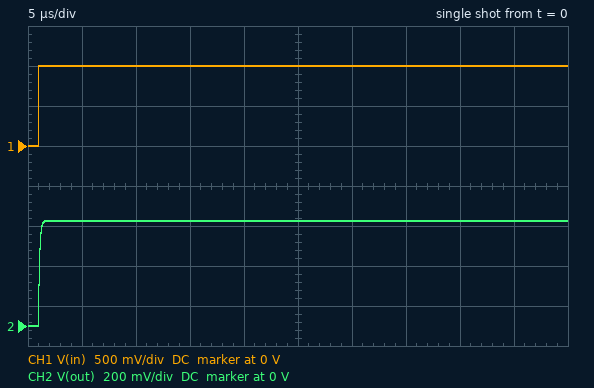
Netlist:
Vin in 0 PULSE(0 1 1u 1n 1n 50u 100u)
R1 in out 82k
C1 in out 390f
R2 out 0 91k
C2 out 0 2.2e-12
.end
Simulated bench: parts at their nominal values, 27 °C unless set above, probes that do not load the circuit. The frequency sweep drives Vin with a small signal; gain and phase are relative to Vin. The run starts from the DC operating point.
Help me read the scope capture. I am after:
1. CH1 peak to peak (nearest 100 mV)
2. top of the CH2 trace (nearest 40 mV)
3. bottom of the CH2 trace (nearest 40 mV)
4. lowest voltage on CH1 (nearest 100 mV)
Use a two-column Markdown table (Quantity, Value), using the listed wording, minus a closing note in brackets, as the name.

| Quantity | Value |
|---|---|
| CH1 peak to peak | 1.0 V |
| top of the CH2 trace | 520 mV |
| bottom of the CH2 trace | 0 V |
| lowest voltage on CH1 | 0 V |
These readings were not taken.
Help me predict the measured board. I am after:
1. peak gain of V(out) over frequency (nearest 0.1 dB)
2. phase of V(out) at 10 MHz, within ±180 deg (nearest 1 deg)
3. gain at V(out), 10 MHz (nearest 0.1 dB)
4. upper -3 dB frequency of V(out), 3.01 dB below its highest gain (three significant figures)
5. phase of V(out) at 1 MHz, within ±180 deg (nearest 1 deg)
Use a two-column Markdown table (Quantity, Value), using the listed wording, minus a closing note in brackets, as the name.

| Quantity | Value |
|---|---|
| peak gain of V(out) over frequency | -5.6 dB |
| phase of V(out) at 10 MHz, within ±180 deg | -18 deg |
| gain at V(out), 10 MHz | -15.6 dB |
| upper -3 dB frequency of V(out), 3.01 dB below its highest gain | 1.56 MHz |
| phase of V(out) at 1 MHz, within ±180 deg | -24 deg |
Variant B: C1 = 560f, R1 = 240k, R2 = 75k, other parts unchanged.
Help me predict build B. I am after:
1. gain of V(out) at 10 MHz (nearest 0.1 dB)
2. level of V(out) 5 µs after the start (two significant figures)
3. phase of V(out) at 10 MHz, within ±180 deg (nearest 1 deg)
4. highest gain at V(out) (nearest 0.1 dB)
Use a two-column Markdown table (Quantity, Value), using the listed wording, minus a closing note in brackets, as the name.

| Quantity | Value |
|---|---|
| gain of V(out) at 10 MHz | -13.8 dB |
| level of V(out) 5 µs after the start | 240 mV |
| phase of V(out) at 10 MHz, within ±180 deg | -1 deg |
| highest gain at V(out) | -12.5 dB |
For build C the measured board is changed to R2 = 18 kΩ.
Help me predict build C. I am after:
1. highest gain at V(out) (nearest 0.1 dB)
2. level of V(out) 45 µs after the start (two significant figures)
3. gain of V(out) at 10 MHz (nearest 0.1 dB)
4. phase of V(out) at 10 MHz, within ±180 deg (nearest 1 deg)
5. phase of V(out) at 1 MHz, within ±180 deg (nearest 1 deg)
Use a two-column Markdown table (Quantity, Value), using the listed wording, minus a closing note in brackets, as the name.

| Quantity | Value |
|---|---|
| highest gain at V(out) | -14.9 dB |
| level of V(out) 45 µs after the start | 180 mV |
| gain of V(out) at 10 MHz | -16.2 dB |
| phase of V(out) at 10 MHz, within ±180 deg | -4 deg |
| phase of V(out) at 1 MHz, within ±180 deg | -2 deg |
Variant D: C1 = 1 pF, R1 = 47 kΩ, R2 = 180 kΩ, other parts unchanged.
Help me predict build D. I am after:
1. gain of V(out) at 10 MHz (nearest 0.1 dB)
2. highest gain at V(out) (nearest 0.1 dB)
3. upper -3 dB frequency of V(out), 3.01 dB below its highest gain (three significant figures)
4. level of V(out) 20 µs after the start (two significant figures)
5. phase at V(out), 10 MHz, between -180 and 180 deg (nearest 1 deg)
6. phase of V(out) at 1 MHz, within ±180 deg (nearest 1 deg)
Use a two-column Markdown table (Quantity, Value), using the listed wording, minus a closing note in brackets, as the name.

| Quantity | Value |
|---|---|
| gain of V(out) at 10 MHz | -9.7 dB |
| highest gain at V(out) | -2.0 dB |
| upper -3 dB frequency of V(out), 3.01 dB below its highest gain | 1.61 MHz |
| level of V(out) 20 µs after the start | 790 mV |
| phase at V(out), 10 MHz, between -180 and 180 deg | -11 deg |
| phase of V(out) at 1 MHz, within ±180 deg | -20 deg |
